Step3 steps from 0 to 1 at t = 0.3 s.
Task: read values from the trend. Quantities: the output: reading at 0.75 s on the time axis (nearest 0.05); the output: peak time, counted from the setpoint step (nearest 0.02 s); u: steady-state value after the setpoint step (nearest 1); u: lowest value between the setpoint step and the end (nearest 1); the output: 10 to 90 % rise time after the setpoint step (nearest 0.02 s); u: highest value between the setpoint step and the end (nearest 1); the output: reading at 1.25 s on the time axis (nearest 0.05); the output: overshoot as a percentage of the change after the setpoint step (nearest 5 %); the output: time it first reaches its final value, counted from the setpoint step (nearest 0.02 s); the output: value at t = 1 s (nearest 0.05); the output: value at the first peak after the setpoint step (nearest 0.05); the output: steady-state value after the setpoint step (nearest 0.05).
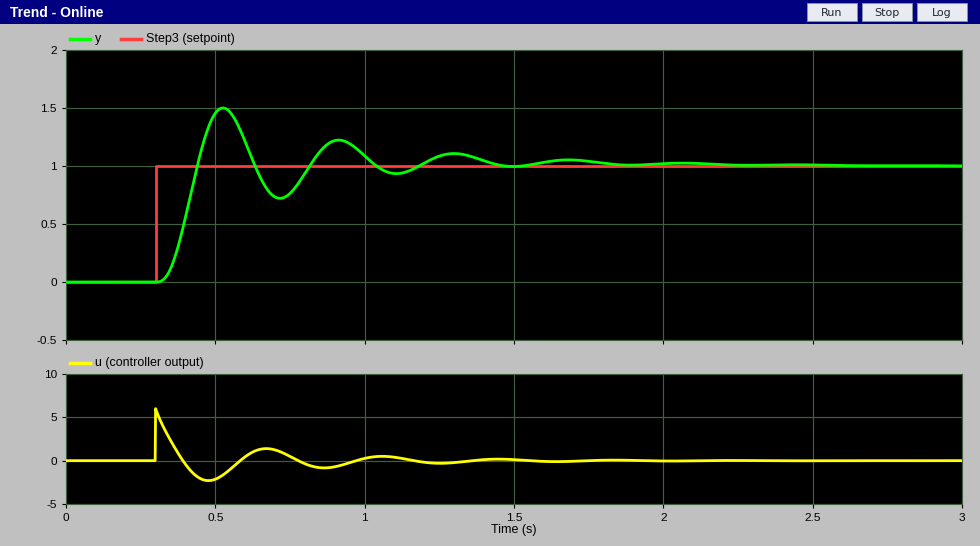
0.75
0.22 s
0
-2
0.08 s
6
1.10
50 %
0.14 s
1.10
1.50
1.00
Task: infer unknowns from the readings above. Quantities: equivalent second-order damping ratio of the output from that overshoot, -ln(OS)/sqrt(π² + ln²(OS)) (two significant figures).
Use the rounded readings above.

0.22
